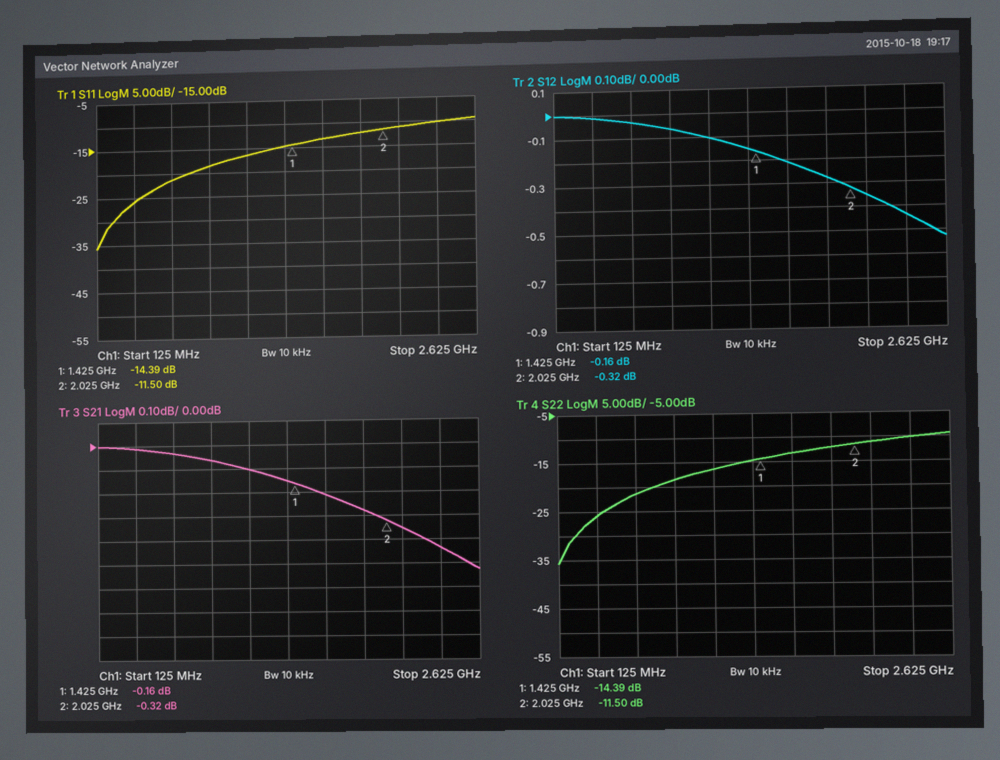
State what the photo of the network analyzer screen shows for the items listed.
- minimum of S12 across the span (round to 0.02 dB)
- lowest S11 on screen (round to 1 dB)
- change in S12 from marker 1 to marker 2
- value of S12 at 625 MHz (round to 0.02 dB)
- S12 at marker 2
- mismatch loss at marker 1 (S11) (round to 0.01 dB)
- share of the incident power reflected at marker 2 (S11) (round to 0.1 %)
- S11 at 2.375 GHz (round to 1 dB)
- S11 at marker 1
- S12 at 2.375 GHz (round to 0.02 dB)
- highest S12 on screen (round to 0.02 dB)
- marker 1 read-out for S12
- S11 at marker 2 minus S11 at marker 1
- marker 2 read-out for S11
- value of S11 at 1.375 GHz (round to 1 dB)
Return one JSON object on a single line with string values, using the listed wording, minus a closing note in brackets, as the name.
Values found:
{"minimum of S12 across the span": "-0.52 dB", "lowest S11 on screen": "-36 dB", "change in S12 from marker 1 to marker 2": "-0.16 dB", "value of S12 at 625 MHz": "-0.04 dB", "S12 at marker 2": "-0.32 dB", "mismatch loss at marker 1 (S11)": "0.16 dB", "share of the incident power reflected at marker 2 (S11)": "7.1 %", "S11 at 2.375 GHz": "-10 dB", "S11 at marker 1": "-14.39 dB", "S12 at 2.375 GHz": "-0.44 dB", "highest S12 on screen": "0.00 dB", "marker 1 read-out for S12": "-0.16 dB", "S11 at marker 2 minus S11 at marker 1": "2.89 dB", "marker 2 read-out for S11": "-11.50 dB", "value of S11 at 1.375 GHz": "-15 dB"}
